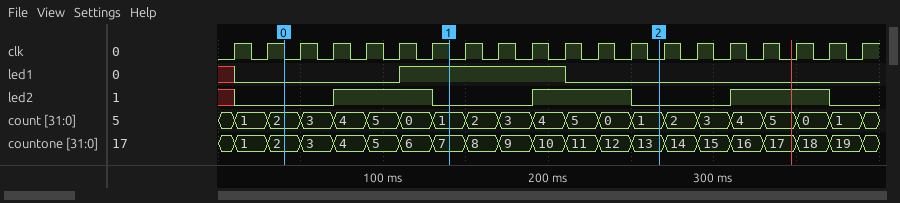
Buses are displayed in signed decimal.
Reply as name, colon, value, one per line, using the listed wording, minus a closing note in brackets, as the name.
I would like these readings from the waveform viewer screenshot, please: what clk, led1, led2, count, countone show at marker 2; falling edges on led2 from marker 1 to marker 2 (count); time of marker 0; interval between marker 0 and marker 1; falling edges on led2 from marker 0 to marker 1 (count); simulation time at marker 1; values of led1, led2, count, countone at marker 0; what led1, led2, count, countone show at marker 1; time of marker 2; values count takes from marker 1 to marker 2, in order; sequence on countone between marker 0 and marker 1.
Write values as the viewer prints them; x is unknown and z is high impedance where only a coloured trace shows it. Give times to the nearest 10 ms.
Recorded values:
what clk, led1, led2, count, countone show at marker 2: clk=0, led1=0, led2=0, count=1, countone=13
falling edges on led2 from marker 1 to marker 2: 1
time of marker 0: 40 ms
interval between marker 0 and marker 1: 100 ms
falling edges on led2 from marker 0 to marker 1: 1
simulation time at marker 1: 140 ms
values of led1, led2, count, countone at marker 0: led1=0, led2=0, count=2, countone=2
what led1, led2, count, countone show at marker 1: led1=1, led2=0, count=1, countone=7
time of marker 2: 270 ms
values count takes from marker 1 to marker 2, in order: 1, 2, 3, 4, 5, 0, 1
sequence on countone between marker 0 and marker 1: 2, 3, 4, 5, 6, 7
